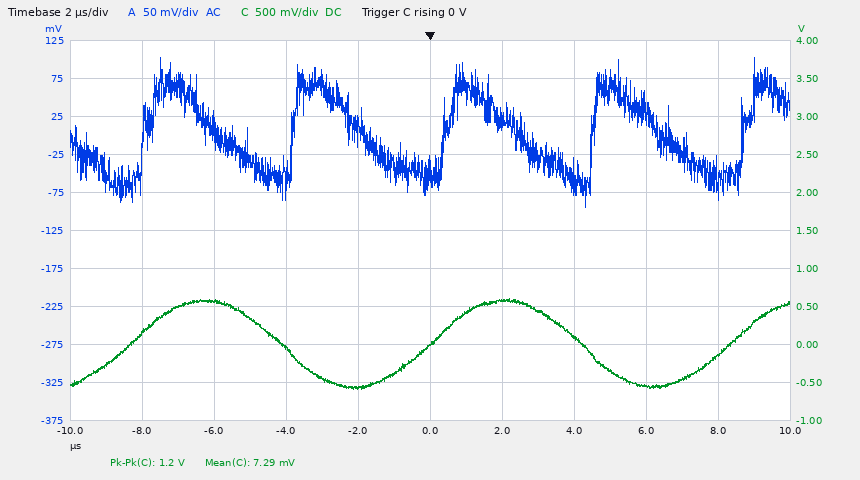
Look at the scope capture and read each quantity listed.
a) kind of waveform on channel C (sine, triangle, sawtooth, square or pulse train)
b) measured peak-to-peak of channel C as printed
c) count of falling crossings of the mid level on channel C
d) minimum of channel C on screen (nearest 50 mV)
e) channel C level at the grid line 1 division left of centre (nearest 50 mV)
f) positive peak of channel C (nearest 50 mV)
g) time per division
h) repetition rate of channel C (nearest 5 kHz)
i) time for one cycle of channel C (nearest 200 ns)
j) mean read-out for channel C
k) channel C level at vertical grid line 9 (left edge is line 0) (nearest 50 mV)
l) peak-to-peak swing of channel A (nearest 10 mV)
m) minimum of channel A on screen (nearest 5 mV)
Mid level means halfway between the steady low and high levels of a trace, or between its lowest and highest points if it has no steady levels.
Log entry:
sine
1.2 V
2
-600 mV
-550 mV
600 mV
2 µs
120 kHz
8.4 µs
7.29 mV
-150 mV
200 mV
-95 mV
